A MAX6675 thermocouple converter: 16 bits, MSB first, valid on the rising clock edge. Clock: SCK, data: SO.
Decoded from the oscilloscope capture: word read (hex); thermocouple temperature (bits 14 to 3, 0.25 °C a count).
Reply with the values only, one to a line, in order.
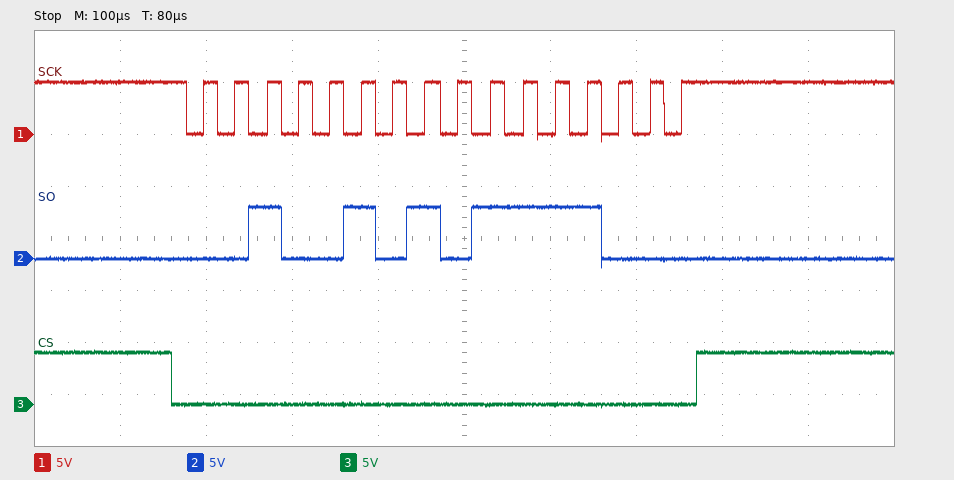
0x2578
299.75 °C
